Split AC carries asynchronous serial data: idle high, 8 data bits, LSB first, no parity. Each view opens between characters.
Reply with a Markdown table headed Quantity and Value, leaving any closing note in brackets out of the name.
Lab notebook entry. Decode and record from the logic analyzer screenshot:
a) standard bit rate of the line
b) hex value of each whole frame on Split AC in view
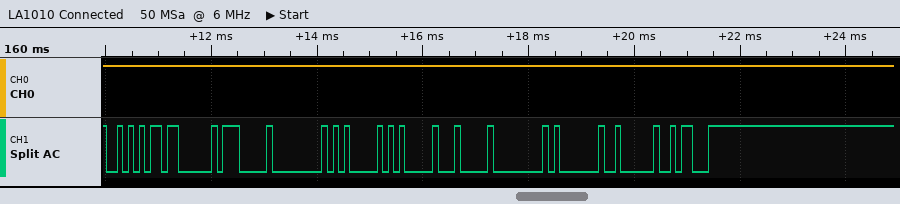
| Quantity | Value |
|---|---|
| standard bit rate of the line | 9600 baud |
| hex value of each whole frame on Split AC in view | AA, 03, 07, 00, 05, 05, 04, 00, 01, 02, 1A |
